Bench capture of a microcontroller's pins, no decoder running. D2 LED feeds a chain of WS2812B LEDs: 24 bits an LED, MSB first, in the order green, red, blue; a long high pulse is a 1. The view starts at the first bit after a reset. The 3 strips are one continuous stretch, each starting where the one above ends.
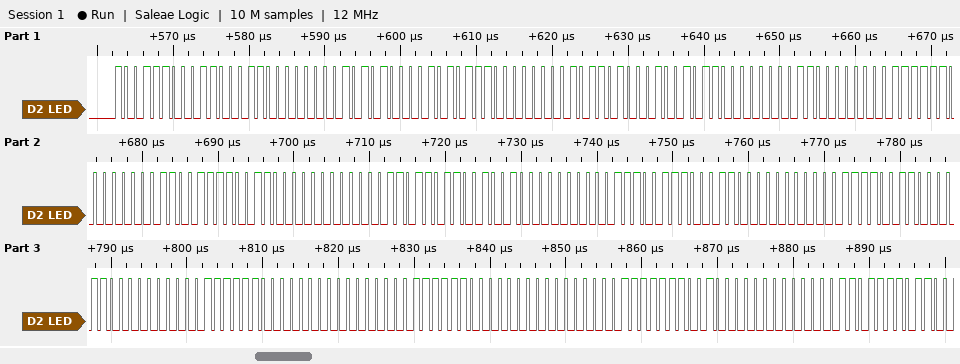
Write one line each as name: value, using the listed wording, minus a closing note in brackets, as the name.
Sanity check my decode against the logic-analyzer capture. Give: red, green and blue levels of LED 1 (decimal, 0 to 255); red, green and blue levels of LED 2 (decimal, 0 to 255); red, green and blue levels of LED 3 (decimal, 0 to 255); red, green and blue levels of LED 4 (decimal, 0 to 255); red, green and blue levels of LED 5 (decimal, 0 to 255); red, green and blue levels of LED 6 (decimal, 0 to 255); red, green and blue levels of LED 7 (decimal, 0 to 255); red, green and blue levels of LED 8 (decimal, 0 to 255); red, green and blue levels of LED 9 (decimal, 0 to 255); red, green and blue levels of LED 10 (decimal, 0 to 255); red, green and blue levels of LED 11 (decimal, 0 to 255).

red, green and blue levels of LED 1: 99, 156, 0
red, green and blue levels of LED 2: 87, 168, 0
red, green and blue levels of LED 3: 75, 180, 0
red, green and blue levels of LED 4: 63, 192, 0
red, green and blue levels of LED 5: 48, 207, 0
red, green and blue levels of LED 6: 36, 219, 0
red, green and blue levels of LED 7: 24, 231, 0
red, green and blue levels of LED 8: 12, 243, 0
red, green and blue levels of LED 9: 0, 252, 3
red, green and blue levels of LED 10: 0, 240, 15
red, green and blue levels of LED 11: 0, 228, 27
